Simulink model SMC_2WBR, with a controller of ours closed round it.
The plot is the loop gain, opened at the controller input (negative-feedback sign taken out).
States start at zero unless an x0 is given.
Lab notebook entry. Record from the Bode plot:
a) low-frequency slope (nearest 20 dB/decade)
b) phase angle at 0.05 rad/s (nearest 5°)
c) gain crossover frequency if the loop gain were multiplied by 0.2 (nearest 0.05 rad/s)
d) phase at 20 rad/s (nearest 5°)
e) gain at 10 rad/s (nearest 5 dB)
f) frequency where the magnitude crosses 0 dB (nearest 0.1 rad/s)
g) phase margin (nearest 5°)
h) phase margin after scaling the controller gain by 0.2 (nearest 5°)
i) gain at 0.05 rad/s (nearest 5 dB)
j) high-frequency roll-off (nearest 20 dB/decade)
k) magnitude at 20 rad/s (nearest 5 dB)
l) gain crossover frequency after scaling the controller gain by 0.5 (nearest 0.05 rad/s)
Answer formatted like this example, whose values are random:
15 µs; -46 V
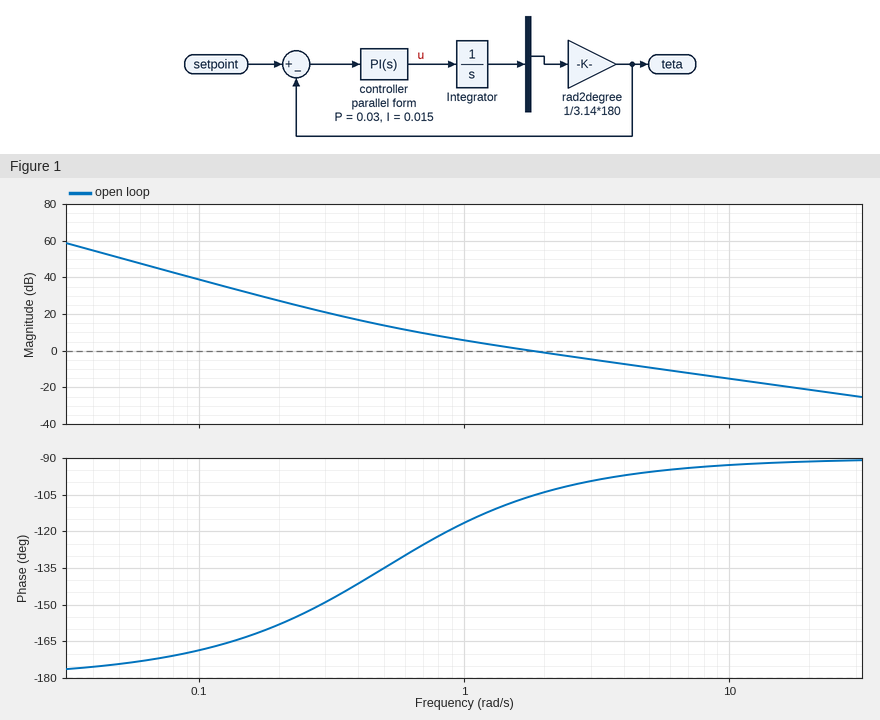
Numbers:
-40 dB/decade; -175°; 0.50 rad/s; -90°; -15 dB; 1.8 rad/s; 75°; 45°; 50 dB; -20 dB/decade; -20 dB; 0.95 rad/s
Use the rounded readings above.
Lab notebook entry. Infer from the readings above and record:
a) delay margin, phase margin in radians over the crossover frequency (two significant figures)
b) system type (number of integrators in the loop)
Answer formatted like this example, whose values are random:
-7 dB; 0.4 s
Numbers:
0.73 s; 2
